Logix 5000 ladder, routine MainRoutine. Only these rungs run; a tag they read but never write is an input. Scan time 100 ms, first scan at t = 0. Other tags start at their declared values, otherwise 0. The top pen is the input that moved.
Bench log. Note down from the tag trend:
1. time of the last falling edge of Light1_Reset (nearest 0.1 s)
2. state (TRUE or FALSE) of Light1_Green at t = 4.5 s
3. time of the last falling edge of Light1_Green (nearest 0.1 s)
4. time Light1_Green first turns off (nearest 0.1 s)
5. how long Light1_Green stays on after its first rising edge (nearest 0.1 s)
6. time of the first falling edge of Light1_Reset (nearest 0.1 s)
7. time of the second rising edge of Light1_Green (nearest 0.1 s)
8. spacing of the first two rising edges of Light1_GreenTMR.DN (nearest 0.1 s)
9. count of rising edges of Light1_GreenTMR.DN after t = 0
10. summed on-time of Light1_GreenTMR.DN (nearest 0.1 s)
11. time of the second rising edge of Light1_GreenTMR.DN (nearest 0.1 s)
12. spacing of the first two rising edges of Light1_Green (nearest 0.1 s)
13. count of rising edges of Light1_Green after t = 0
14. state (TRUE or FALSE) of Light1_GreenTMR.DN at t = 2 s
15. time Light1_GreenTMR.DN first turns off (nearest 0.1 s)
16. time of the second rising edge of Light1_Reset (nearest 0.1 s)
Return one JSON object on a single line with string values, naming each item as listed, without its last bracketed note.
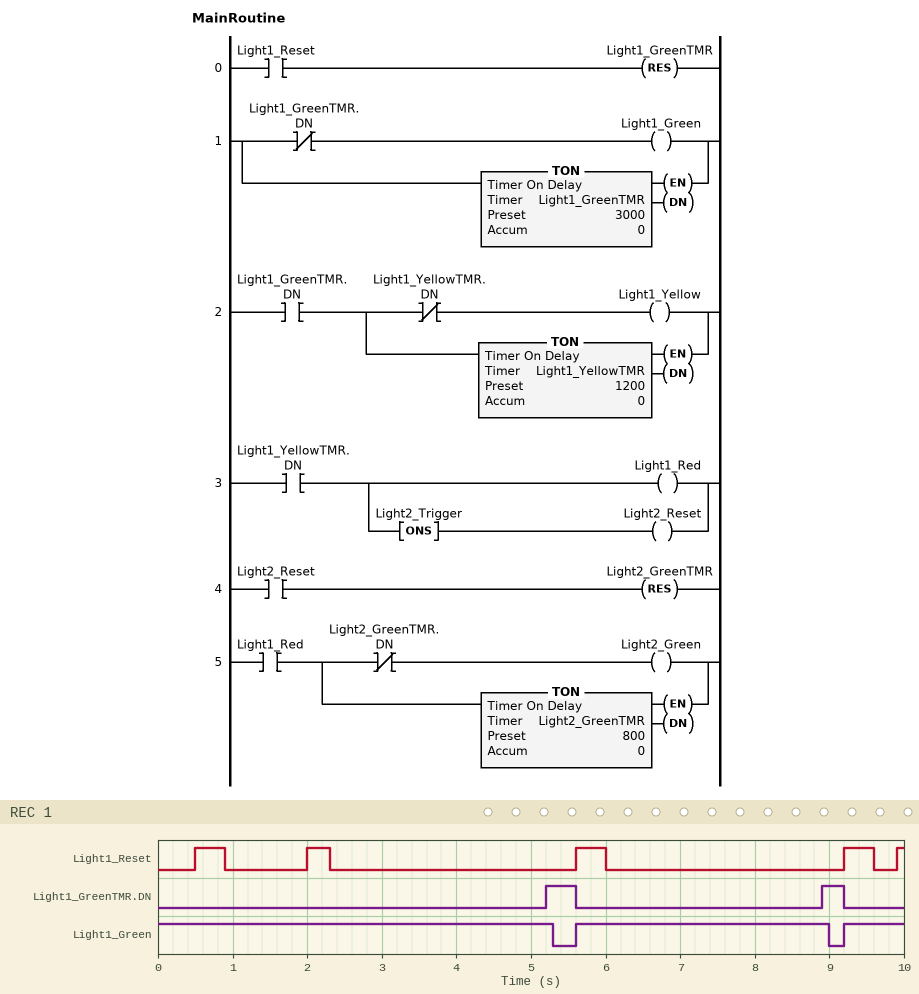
{"time of the last falling edge of Light1_Reset": "9.6 s", "state (TRUE or FALSE) of Light1_Green at t = 4.5 s": "TRUE", "time of the last falling edge of Light1_Green": "9.0 s", "time Light1_Green first turns off": "5.3 s", "how long Light1_Green stays on after its first rising edge": "3.4 s", "time of the first falling edge of Light1_Reset": "0.9 s", "time of the second rising edge of Light1_Green": "9.2 s", "spacing of the first two rising edges of Light1_GreenTMR.DN": "3.7 s", "count of rising edges of Light1_GreenTMR.DN after t = 0": "2", "summed on-time of Light1_GreenTMR.DN": "0.7 s", "time of the second rising edge of Light1_GreenTMR.DN": "8.9 s", "spacing of the first two rising edges of Light1_Green": "3.6 s", "count of rising edges of Light1_Green after t = 0": "2", "state (TRUE or FALSE) of Light1_GreenTMR.DN at t = 2 s": "FALSE", "time Light1_GreenTMR.DN first turns off": "5.6 s", "time of the second rising edge of Light1_Reset": "2.0 s"}
